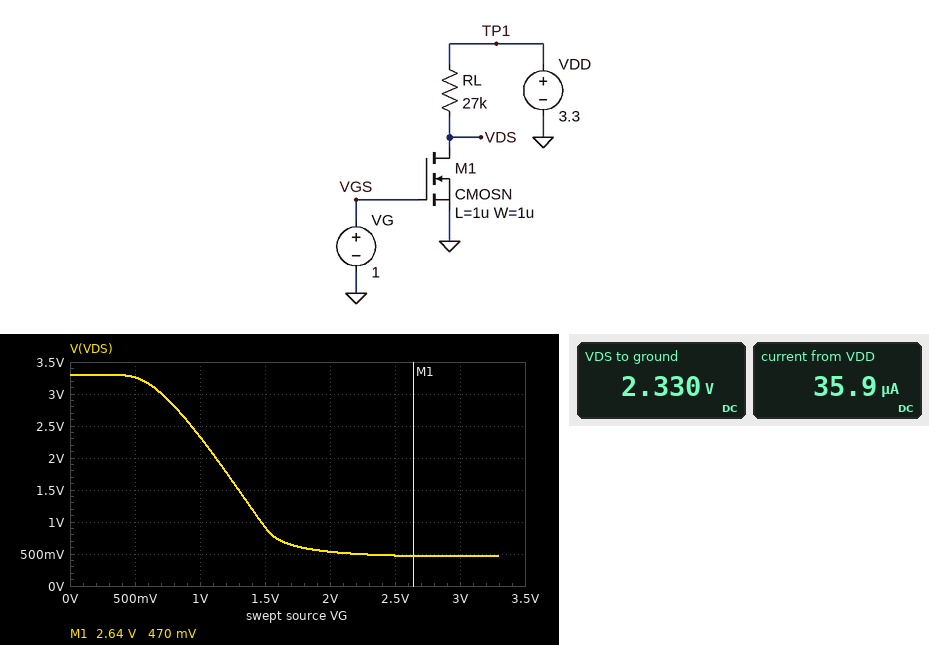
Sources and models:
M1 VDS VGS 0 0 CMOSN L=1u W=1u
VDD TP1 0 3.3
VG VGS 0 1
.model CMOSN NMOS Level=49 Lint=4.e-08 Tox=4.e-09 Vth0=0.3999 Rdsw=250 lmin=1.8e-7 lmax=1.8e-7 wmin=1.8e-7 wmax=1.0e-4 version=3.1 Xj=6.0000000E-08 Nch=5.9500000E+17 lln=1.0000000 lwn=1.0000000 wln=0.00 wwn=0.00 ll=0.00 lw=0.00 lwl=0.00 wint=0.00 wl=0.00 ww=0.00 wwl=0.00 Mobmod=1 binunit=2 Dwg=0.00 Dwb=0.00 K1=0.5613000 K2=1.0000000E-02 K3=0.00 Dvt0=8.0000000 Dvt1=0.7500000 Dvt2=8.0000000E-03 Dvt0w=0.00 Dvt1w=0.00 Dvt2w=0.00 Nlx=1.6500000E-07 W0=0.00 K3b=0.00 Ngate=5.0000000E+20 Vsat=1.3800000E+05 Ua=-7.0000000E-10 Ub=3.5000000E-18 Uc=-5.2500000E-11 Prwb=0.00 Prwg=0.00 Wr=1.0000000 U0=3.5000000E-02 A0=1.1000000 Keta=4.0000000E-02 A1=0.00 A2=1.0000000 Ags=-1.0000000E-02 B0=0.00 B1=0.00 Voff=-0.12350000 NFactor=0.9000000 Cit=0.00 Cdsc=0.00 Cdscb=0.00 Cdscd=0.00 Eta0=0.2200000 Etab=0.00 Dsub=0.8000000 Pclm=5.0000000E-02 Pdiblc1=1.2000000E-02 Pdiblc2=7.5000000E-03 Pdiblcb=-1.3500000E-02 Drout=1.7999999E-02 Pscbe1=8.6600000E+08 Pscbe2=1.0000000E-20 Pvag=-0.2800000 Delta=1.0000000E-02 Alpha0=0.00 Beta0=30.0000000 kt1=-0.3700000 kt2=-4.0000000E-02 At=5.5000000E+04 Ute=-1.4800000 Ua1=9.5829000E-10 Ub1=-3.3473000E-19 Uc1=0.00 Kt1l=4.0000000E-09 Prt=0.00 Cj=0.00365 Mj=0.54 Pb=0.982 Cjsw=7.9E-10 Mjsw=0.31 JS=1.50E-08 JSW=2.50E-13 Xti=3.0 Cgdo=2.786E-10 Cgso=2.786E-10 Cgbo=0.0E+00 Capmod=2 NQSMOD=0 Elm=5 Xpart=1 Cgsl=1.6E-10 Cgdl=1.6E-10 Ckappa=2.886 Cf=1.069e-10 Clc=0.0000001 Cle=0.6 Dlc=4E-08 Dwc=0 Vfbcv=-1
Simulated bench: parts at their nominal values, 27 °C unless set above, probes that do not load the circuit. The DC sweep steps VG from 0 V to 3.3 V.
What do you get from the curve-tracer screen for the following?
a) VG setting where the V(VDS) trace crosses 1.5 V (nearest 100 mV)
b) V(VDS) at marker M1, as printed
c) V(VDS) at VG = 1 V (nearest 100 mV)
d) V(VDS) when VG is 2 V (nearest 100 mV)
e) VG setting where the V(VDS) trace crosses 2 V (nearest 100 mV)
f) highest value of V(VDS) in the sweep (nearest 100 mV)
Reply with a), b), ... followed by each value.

a) 1.3 V
b) 470 mV
c) 2.3 V
d) 500 mV
e) 1.1 V
f) 3.3 V
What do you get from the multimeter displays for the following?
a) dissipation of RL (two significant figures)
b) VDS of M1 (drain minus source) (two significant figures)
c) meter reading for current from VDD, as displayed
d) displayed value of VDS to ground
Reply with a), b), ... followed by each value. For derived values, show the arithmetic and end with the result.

a) (3.3 V - 2.33 V)^2 / 27 kΩ = 35 µW
b) 2.33 V = 2.3 V
c) 35.9 µA
d) 2.330 V
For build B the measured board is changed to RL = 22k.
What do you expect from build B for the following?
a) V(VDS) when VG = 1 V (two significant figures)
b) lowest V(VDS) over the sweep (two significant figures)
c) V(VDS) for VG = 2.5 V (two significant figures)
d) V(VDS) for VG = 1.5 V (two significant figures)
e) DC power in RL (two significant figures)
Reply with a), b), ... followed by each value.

a) 2.5 V
b) 560 mV
c) 590 mV
d) 1.3 V
e) 29 µW
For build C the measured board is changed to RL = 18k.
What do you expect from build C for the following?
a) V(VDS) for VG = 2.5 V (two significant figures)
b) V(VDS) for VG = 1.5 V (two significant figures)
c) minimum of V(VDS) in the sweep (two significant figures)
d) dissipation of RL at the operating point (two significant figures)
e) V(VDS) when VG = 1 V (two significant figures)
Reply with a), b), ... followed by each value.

a) 720 mV
b) 1.7 V
c) 680 mV
d) 24 µW
e) 2.6 V
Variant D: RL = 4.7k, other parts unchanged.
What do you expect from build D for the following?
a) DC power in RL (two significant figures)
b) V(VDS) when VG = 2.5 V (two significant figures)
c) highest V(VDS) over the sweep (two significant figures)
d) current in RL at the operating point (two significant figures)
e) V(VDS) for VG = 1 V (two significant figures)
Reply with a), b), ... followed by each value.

a) 6.6 µW
b) 2.3 V
c) 3.3 V
d) 37 µA
e) 3.1 V
